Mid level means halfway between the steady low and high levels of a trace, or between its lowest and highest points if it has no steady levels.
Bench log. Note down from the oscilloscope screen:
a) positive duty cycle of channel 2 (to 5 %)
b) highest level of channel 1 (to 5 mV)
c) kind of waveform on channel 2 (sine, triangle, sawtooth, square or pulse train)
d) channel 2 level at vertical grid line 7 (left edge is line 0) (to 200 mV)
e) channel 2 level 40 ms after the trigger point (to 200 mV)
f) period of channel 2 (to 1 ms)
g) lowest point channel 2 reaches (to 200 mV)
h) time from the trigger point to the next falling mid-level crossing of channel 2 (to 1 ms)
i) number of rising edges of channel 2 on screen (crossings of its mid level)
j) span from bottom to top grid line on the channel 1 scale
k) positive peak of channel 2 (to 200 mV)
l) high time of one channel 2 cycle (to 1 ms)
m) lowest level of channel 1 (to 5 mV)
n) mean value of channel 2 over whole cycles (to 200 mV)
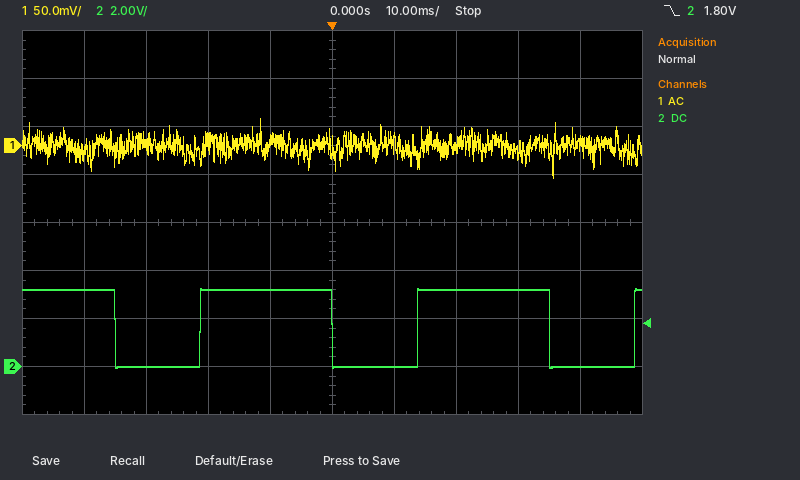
60 %
30 mV
pulse train
3.2 V
0.0 V
35 ms
0.0 V
35 ms
3
400 mV
3.2 V
21 ms
-35 mV
2.0 V
